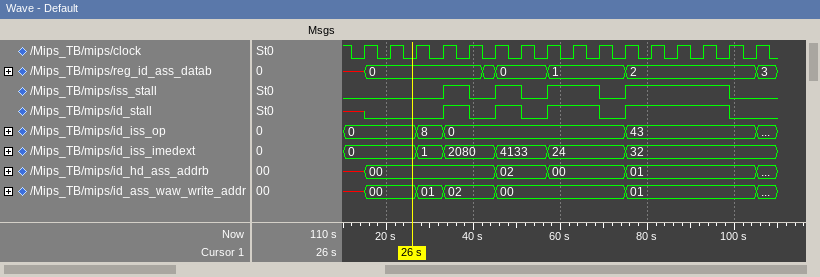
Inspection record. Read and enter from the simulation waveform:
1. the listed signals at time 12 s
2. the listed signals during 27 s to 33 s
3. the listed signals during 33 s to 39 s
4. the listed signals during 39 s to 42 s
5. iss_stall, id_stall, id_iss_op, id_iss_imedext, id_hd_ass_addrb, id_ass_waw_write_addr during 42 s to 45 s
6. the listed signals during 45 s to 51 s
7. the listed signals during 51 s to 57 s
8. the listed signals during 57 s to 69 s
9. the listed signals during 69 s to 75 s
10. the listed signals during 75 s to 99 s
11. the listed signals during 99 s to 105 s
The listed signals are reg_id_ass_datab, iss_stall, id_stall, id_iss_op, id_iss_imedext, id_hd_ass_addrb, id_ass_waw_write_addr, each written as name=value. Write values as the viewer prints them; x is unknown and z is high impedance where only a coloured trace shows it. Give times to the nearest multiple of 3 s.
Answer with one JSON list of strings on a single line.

["reg_id_ass_datab=x, iss_stall=0, id_stall=x, id_iss_op=0, id_iss_imedext=0, id_hd_ass_addrb=x, id_ass_waw_write_addr=x", "reg_id_ass_datab=0, iss_stall=0, id_stall=0, id_iss_op=8, id_iss_imedext=1, id_hd_ass_addrb=00, id_ass_waw_write_addr=01", "reg_id_ass_datab=0, iss_stall=1, id_stall=1, id_iss_op=0, id_iss_imedext=2080, id_hd_ass_addrb=00, id_ass_waw_write_addr=02", "reg_id_ass_datab=0, iss_stall=0, id_stall=0, id_iss_op=0, id_iss_imedext=2080, id_hd_ass_addrb=00, id_ass_waw_write_addr=02", "iss_stall=0, id_stall=0, id_iss_op=0, id_iss_imedext=2080, id_hd_ass_addrb=00, id_ass_waw_write_addr=02", "reg_id_ass_datab=0, iss_stall=1, id_stall=1, id_iss_op=0, id_iss_imedext=4133, id_hd_ass_addrb=02, id_ass_waw_write_addr=00", "reg_id_ass_datab=0, iss_stall=0, id_stall=0, id_iss_op=0, id_iss_imedext=4133, id_hd_ass_addrb=02, id_ass_waw_write_addr=00", "reg_id_ass_datab=1, iss_stall=1, id_stall=1, id_iss_op=0, id_iss_imedext=24, id_hd_ass_addrb=00, id_ass_waw_write_addr=00", "reg_id_ass_datab=1, iss_stall=0, id_stall=0, id_iss_op=0, id_iss_imedext=24, id_hd_ass_addrb=00, id_ass_waw_write_addr=00", "reg_id_ass_datab=2, iss_stall=1, id_stall=1, id_iss_op=43, id_iss_imedext=32, id_hd_ass_addrb=01, id_ass_waw_write_addr=01", "reg_id_ass_datab=2, iss_stall=0, id_stall=0, id_iss_op=43, id_iss_imedext=32, id_hd_ass_addrb=01, id_ass_waw_write_addr=01"]
